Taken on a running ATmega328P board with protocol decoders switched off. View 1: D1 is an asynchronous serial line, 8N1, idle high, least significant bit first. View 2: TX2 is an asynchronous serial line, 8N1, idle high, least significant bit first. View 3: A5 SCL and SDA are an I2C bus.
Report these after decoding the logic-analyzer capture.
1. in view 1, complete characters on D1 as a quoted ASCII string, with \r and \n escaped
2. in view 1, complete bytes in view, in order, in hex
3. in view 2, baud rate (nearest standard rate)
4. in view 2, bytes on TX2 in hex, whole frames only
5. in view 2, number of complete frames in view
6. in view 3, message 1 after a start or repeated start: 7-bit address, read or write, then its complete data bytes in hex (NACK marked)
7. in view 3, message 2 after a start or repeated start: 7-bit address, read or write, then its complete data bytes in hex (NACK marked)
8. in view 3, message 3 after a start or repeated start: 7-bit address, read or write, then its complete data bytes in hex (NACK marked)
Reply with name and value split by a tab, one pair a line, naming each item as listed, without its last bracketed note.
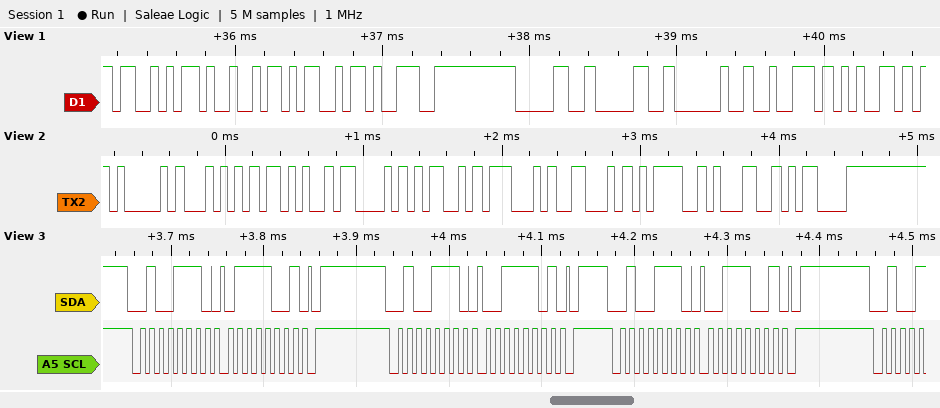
in view 1, complete characters on D1 as a quoted ASCII string, with \r and \n escaped	"SIM900 re"
in view 1, complete bytes in view, in order, in hex	53 49 4D 39 30 30 20 72 65
in view 2, baud rate	19200 baud
in view 2, bytes on TX2 in hex, whole frames only	0x41 0x54 0x2B 0x43 0x4D 0x47 0x46 0x3D 0x31 0x0D
in view 2, number of complete frames in view	10
in view 3, message 1 after a start or repeated start: 7-bit address, read or write, then its complete data bytes in hex	0x27 write: 79
in view 3, message 2 after a start or repeated start: 7-bit address, read or write, then its complete data bytes in hex	0x27 write: 3D
in view 3, message 3 after a start or repeated start: 7-bit address, read or write, then its complete data bytes in hex	0x27 write: 39
